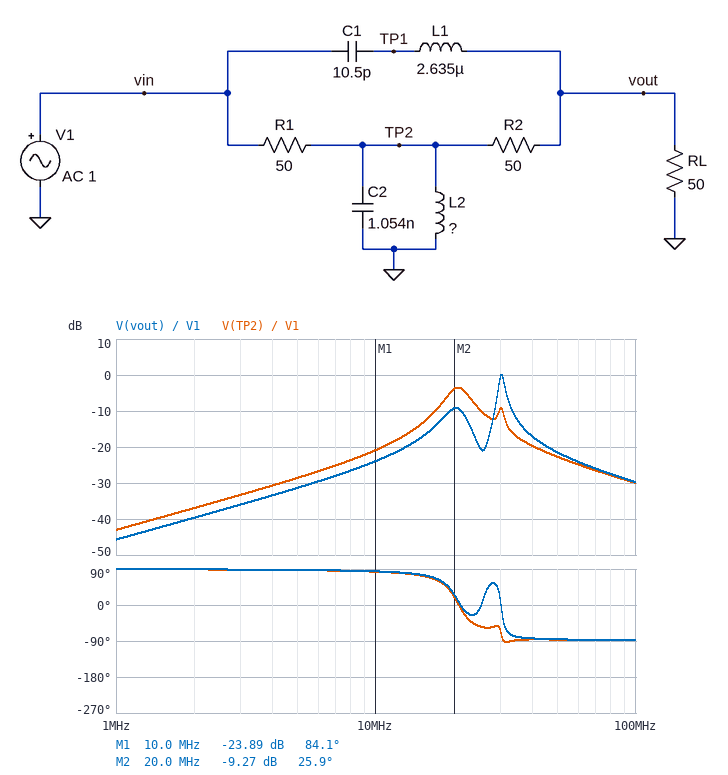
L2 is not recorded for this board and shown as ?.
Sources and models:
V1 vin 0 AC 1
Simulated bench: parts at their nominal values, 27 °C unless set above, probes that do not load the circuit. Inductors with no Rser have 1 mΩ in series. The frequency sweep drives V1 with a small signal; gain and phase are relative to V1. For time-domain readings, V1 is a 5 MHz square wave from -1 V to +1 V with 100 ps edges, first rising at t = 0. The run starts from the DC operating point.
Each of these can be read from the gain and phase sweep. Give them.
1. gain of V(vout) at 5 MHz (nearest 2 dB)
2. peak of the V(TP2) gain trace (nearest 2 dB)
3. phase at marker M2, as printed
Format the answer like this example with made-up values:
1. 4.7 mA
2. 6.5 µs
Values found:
1. -32 dB
2. -4 dB
3. 25.9 deg
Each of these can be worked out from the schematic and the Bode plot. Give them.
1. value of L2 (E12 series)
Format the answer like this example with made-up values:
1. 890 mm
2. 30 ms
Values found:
1. 56 nH
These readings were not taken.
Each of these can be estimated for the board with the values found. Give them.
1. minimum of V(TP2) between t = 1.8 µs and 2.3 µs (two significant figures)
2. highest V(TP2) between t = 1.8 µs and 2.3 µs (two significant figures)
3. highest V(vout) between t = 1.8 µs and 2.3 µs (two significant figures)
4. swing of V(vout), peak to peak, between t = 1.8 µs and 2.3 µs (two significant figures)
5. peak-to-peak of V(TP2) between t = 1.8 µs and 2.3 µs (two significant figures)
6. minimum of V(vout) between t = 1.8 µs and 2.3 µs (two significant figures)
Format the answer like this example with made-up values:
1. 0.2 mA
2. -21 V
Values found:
1. -210 mV
2. 210 mV
3. 150 mV
4. 310 mV
5. 410 mV
6. -150 mV
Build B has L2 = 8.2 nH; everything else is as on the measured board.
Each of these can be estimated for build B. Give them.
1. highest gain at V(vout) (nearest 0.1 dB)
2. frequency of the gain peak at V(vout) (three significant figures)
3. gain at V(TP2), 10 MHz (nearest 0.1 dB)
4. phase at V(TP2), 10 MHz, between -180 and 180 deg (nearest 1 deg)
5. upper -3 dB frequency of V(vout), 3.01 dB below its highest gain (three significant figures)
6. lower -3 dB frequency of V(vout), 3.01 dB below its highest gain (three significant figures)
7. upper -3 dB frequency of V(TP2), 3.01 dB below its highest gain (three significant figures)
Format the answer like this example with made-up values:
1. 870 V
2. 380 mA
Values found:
1. 0 dB
2. 30.2 MHz
3. -39.4 dB
4. 90 deg
5. 31.0 MHz
6. 29.5 MHz
7. 56.5 MHz
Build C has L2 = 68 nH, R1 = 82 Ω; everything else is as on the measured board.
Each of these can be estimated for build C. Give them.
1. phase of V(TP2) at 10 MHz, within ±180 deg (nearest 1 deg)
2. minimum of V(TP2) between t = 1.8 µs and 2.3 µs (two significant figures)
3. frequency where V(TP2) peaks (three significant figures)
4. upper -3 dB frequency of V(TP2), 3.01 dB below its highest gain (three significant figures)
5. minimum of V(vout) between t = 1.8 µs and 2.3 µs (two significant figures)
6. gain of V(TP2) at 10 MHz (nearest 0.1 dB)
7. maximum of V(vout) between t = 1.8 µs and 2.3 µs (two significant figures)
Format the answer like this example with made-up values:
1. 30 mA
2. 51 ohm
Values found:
1. 84 deg
2. -140 mV
3. 18.8 MHz
4. 20.5 MHz
5. -130 mV
6. -22.8 dB
7. 130 mV
